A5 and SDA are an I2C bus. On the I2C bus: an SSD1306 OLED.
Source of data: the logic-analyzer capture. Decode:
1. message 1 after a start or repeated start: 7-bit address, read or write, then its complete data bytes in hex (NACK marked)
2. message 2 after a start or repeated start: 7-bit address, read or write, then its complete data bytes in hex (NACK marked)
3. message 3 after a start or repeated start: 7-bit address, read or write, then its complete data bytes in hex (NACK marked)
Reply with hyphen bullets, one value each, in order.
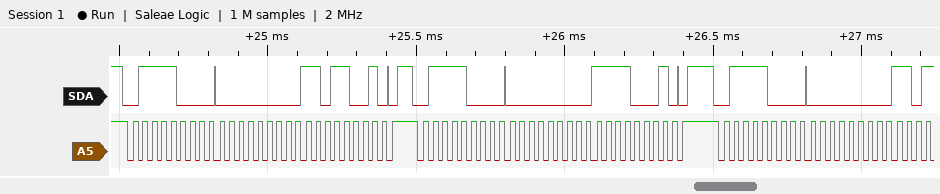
- 0x3C write: 00 D9
- 0x3C write: 00 F1
- 0x3C write: 00
